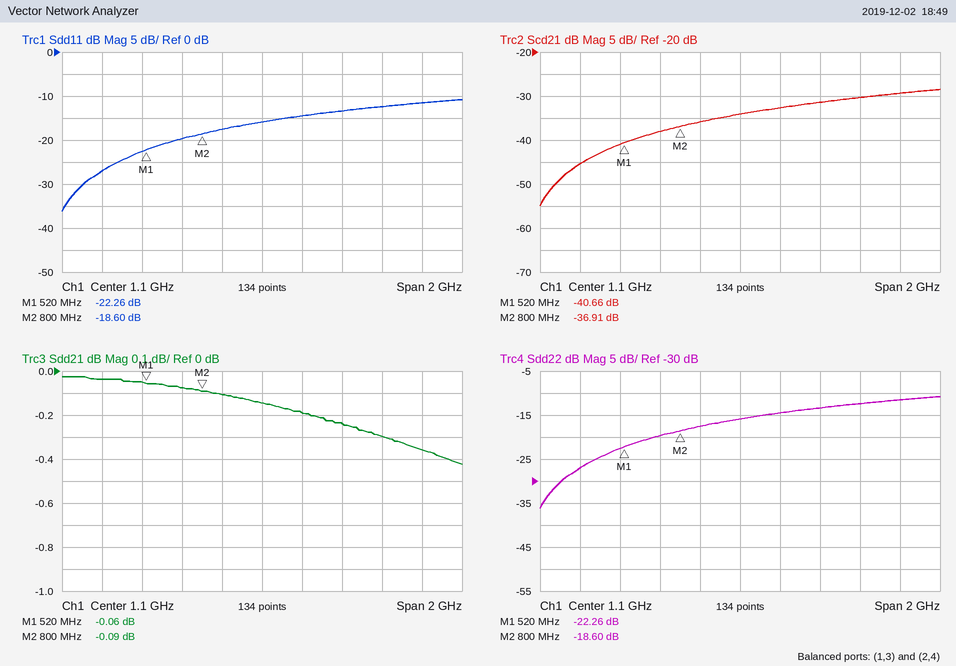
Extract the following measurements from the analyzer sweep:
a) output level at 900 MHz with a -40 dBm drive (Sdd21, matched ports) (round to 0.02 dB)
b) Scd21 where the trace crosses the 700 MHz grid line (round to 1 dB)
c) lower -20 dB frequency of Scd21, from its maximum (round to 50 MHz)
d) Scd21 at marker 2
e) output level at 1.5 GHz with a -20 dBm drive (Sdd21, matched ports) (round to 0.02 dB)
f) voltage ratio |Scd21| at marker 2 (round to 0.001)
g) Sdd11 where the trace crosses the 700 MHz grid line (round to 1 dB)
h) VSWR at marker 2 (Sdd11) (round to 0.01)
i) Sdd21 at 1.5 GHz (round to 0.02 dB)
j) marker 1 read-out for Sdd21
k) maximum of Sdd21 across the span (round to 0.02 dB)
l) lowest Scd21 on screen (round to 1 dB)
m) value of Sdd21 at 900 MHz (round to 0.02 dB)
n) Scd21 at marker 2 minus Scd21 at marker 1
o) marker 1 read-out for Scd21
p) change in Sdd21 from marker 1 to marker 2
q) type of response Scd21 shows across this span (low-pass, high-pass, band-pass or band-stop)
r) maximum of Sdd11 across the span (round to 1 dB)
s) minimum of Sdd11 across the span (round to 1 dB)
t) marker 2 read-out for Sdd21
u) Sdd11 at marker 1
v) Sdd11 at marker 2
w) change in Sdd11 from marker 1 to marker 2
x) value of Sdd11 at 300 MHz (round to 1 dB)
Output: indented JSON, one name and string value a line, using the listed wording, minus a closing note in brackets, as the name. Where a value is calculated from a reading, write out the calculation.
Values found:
{
  "output level at 900 MHz with a -40 dBm drive (Sdd21, matched ports)": "-40 dBm + (-0.10 dB) = -40.10 dBm",
  "Scd21 where the trace crosses the 700 MHz grid line": "-38 dB",
  "lower -20 dB frequency of Scd21, from its maximum": "200 MHz",
  "Scd21 at marker 2": "-36.91 dB",
  "output level at 1.5 GHz with a -20 dBm drive (Sdd21, matched ports)": "-20 dBm + (-0.24 dB) = -20.24 dBm",
  "voltage ratio |Scd21| at marker 2": "10^(-36.91/20) ≈ 0.014",
  "Sdd11 where the trace crosses the 700 MHz grid line": "-20 dB",
  "VSWR at marker 2 (Sdd11)": "(1 + 0.1175)/(1 − 0.1175) ≈ 1.27",
  "Sdd21 at 1.5 GHz": "-0.24 dB",
  "marker 1 read-out for Sdd21": "-0.06 dB",
  "maximum of Sdd21 across the span": "-0.02 dB",
  "lowest Scd21 on screen": "-55 dB",
  "value of Sdd21 at 900 MHz": "-0.10 dB",
  "Scd21 at marker 2 minus Scd21 at marker 1": "-36.91 − (-40.66) = 3.75 dB",
  "marker 1 read-out for Scd21": "-40.66 dB",
  "change in Sdd21 from marker 1 to marker 2": "-0.09 − (-0.06) = -0.03 dB",
  "type of response Scd21 shows across this span": "high-pass",
  "maximum of Sdd11 across the span": "-11 dB",
  "minimum of Sdd11 across the span": "-36 dB",
  "marker 2 read-out for Sdd21": "-0.09 dB",
  "Sdd11 at marker 1": "-22.26 dB",
  "Sdd11 at marker 2": "-18.60 dB",
  "change in Sdd11 from marker 1 to marker 2": "-18.6 − (-22.26) = 3.66 dB",
  "value of Sdd11 at 300 MHz": "-27 dB"
}
